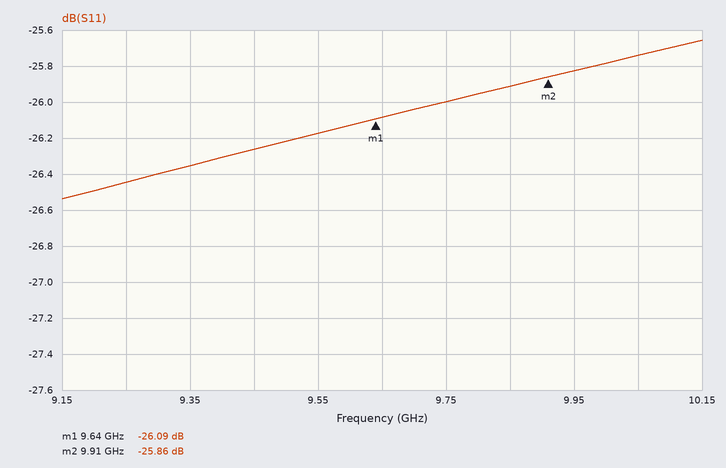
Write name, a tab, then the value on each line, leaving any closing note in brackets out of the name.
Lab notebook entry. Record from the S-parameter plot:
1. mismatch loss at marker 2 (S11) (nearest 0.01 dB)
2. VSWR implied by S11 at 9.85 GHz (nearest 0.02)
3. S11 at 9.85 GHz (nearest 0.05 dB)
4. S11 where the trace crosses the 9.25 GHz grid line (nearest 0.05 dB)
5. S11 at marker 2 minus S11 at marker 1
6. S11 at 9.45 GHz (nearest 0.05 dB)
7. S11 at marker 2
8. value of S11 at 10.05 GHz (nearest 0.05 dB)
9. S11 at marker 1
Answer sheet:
mismatch loss at marker 2 (S11)	0.01 dB
VSWR implied by S11 at 9.85 GHz	1.10
S11 at 9.85 GHz	-25.90 dB
S11 where the trace crosses the 9.25 GHz grid line	-26.45 dB
S11 at marker 2 minus S11 at marker 1	0.23 dB
S11 at 9.45 GHz	-26.25 dB
S11 at marker 2	-25.86 dB
value of S11 at 10.05 GHz	-25.75 dB
S11 at marker 1	-26.09 dB
